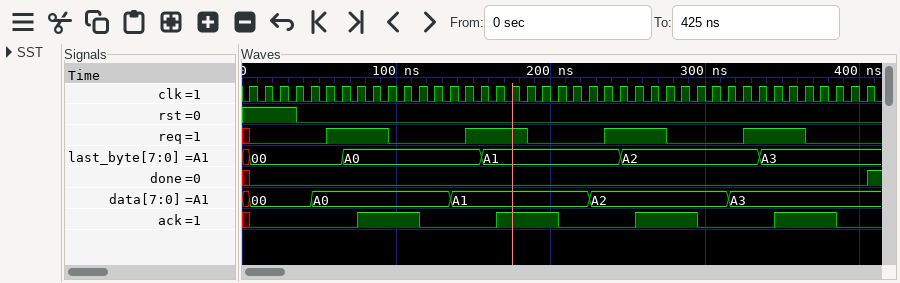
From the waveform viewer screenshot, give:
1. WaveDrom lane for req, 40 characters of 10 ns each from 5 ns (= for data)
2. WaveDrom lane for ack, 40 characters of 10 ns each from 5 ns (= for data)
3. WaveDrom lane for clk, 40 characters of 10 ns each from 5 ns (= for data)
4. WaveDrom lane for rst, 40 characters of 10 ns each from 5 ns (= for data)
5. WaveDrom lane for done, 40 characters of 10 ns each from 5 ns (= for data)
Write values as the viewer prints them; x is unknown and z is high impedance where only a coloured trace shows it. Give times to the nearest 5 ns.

{name: 'req', wave: '0....1...0....1...0....1...0....1...0...'}
{name: 'ack', wave: '0......1...0....1...0....1...0....1...0.'}
{name: 'clk', wave: 'p.......................................'}
{name: 'rst', wave: '1..0....................................'}
{name: 'done', wave: '0.......................................'}
